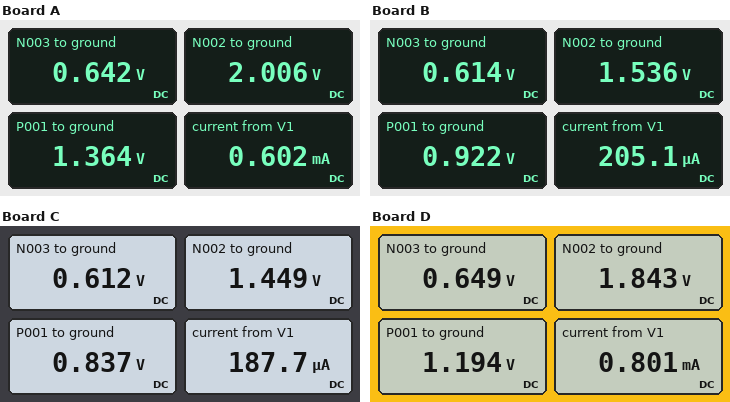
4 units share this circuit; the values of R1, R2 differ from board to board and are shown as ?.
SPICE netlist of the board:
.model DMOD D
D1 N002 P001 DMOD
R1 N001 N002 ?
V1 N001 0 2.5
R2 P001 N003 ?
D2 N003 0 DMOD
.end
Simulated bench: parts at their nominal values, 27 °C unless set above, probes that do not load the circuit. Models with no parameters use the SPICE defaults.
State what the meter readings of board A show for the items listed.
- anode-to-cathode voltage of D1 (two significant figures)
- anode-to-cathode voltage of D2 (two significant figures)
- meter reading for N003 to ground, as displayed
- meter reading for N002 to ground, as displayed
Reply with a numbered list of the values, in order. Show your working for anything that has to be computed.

1. 2.006 V - 1.364 V = 640 mV
2. 642 mV = 640 mV
3. 0.642 V
4. 2.006 V
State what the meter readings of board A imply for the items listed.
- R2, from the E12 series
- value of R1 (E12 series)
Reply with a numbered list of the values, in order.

1. 1.2 kΩ
2. 820 Ω
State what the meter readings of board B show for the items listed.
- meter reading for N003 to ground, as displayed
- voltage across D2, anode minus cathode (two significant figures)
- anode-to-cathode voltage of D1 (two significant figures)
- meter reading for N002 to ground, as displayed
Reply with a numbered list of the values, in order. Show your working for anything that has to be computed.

1. 0.614 V
2. 614 mV = 610 mV
3. 1.536 V - 922 mV = 610 mV
4. 1.536 V
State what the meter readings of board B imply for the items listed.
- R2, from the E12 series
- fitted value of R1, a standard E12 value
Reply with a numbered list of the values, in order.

1. 1.5 kΩ
2. 4.7 kΩ
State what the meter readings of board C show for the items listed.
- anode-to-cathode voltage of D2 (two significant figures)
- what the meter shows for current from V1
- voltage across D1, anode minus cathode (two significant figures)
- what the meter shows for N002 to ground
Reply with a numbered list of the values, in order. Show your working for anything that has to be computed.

1. 612 mV = 610 mV
2. 187.7 µA
3. 1.449 V - 837 mV = 610 mV
4. 1.449 V
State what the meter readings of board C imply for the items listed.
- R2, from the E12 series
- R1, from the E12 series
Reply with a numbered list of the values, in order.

1. 1.2 kΩ
2. 5.6 kΩ
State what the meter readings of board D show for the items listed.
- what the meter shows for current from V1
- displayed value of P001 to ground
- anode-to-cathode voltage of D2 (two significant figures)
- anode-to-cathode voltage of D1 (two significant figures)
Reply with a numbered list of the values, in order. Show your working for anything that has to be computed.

1. 0.801 mA
2. 1.194 V
3. 649 mV = 650 mV
4. 1.843 V - 1.194 V = 650 mV
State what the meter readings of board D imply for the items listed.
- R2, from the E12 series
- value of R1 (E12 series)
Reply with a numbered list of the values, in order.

1. 680 Ω
2. 820 Ω
